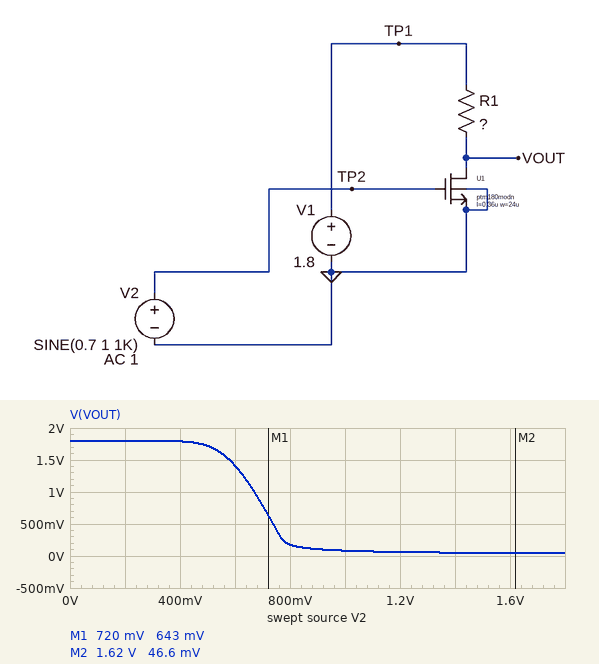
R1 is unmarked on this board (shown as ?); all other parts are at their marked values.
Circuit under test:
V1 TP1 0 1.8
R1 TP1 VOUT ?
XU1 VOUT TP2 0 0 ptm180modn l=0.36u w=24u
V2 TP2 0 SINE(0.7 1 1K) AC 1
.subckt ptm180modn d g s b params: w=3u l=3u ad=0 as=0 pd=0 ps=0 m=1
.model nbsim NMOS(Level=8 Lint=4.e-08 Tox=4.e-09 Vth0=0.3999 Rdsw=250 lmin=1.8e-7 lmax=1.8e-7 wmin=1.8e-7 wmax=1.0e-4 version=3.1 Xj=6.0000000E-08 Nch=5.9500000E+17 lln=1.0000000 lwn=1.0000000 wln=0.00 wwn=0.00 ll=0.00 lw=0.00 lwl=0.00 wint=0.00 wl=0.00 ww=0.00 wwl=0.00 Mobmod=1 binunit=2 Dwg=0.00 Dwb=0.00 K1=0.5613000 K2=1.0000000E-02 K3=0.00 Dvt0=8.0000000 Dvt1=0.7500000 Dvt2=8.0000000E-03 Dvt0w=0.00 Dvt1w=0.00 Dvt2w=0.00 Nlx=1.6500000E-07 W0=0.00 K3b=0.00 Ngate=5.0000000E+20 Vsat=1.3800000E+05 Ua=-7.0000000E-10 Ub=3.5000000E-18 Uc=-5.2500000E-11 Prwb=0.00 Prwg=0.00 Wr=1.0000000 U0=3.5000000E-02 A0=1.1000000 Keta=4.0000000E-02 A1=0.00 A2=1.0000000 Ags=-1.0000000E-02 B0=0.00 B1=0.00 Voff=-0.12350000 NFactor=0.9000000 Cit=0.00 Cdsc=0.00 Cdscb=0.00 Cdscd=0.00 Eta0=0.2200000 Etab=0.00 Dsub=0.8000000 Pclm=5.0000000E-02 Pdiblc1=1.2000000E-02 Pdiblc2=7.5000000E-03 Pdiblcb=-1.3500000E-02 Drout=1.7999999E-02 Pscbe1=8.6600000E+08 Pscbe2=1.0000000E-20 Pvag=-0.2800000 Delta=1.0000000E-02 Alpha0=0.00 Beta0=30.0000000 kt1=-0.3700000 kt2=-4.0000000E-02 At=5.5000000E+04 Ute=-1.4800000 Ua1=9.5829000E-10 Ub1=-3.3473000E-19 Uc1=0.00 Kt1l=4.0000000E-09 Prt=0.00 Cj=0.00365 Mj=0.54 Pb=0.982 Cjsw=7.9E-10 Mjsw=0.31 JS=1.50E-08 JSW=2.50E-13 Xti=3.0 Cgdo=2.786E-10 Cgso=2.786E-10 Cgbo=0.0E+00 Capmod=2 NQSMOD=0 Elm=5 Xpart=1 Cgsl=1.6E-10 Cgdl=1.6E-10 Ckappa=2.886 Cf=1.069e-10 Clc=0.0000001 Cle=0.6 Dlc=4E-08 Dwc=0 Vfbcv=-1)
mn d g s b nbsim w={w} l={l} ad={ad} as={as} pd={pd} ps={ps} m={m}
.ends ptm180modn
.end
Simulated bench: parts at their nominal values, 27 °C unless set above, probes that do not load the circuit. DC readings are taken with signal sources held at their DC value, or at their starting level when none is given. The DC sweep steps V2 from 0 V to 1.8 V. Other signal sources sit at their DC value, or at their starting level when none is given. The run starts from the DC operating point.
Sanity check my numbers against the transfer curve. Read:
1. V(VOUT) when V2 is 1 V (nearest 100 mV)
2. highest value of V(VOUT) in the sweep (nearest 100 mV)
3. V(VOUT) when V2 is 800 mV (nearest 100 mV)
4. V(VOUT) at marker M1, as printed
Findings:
100 mV
1.8 V
200 mV
643 mV
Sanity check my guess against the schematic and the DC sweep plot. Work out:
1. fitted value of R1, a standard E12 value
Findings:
2.7 kΩ
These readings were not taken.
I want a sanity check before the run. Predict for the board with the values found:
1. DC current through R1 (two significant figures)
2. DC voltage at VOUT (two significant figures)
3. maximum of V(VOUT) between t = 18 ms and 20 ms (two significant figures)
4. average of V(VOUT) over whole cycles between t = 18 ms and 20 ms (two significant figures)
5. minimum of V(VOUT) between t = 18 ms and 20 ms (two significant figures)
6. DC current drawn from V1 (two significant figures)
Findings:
370 µA
790 mV
1.8 V
910 mV
45 mV
370 µA
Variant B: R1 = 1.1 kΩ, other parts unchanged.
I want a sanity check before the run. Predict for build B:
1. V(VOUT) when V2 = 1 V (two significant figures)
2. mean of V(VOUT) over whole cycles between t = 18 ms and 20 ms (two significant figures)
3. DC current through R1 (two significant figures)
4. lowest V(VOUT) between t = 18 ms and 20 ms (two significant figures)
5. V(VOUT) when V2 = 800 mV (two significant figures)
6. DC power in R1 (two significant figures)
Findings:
250 mV
1.0 V
410 µA
110 mV
950 mV
190 µW
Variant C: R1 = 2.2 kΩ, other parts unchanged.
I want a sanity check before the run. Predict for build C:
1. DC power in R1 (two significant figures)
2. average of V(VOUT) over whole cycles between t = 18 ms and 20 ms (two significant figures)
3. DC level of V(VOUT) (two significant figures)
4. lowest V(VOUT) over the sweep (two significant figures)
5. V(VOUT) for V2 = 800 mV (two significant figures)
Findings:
330 µW
930 mV
950 mV
54 mV
290 mV
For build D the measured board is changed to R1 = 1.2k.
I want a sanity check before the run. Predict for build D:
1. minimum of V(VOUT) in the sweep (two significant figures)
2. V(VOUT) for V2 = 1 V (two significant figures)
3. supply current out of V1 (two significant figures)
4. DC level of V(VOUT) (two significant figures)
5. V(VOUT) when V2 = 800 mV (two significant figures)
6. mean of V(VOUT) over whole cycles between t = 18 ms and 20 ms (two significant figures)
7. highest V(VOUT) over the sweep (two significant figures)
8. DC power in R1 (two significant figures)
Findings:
99 mV
220 mV
410 µA
1.3 V
880 mV
1.0 V
1.8 V
200 µW
